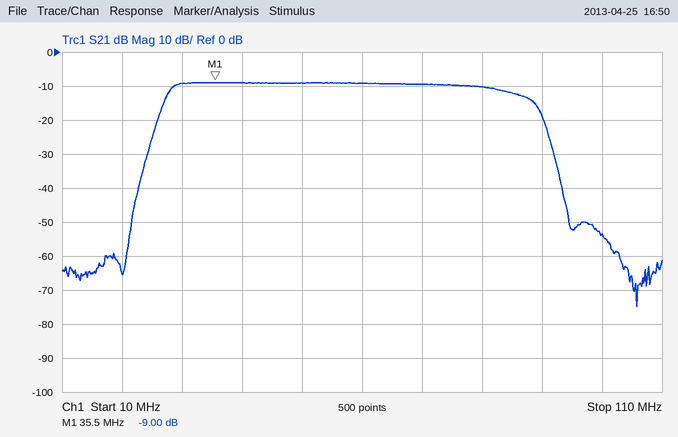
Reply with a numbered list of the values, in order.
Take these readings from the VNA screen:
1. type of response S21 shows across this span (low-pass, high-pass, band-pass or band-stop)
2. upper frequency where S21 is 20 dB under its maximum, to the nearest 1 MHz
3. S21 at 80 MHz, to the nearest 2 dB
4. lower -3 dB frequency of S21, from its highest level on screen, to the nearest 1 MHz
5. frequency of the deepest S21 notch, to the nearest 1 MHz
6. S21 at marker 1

1. band-pass
2. 92 MHz
3. -10 dB
4. 28 MHz
5. 106 MHz
6. -9.00 dB
